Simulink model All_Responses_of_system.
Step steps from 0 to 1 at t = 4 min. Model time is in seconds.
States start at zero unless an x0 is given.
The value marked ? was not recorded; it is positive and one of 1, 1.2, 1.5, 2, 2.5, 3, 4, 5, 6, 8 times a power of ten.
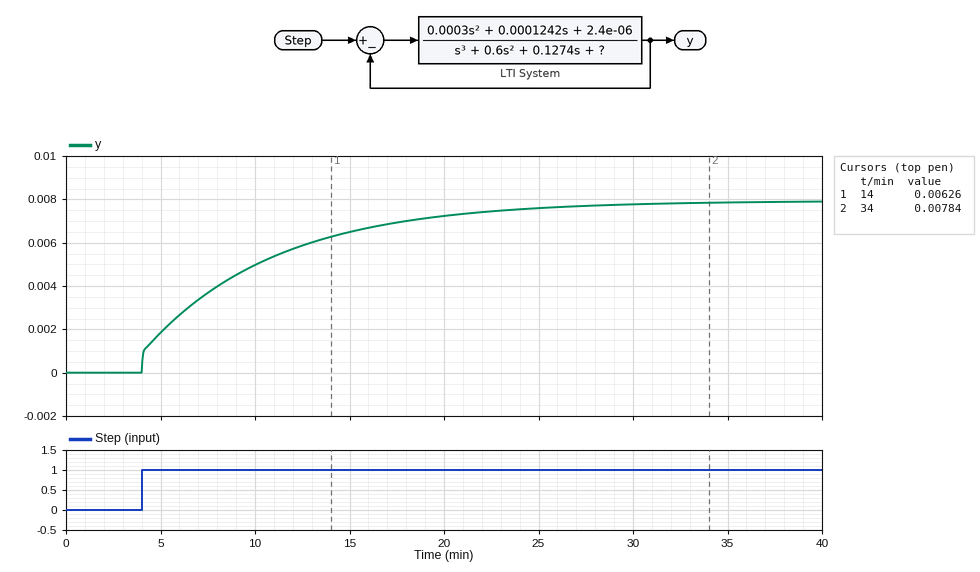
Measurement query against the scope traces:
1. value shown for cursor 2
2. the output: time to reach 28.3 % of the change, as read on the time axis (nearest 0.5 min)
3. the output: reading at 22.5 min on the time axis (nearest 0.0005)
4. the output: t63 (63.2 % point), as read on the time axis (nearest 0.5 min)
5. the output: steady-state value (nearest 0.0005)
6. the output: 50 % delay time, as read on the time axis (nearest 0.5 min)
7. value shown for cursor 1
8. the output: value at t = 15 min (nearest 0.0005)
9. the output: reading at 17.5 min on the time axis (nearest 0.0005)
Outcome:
0.00784
5.5 min
0.0075
10.0 min
0.0080
8.0 min
0.00626
0.0065
0.0070
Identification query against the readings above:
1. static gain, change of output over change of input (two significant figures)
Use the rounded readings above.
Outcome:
0.0080
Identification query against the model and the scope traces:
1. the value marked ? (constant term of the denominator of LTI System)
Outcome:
0.0003
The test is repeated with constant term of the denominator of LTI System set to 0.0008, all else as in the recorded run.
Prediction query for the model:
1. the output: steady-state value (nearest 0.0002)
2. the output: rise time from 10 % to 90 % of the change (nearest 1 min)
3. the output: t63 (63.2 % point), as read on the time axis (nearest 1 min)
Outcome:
0.0030
5 min
6 min
